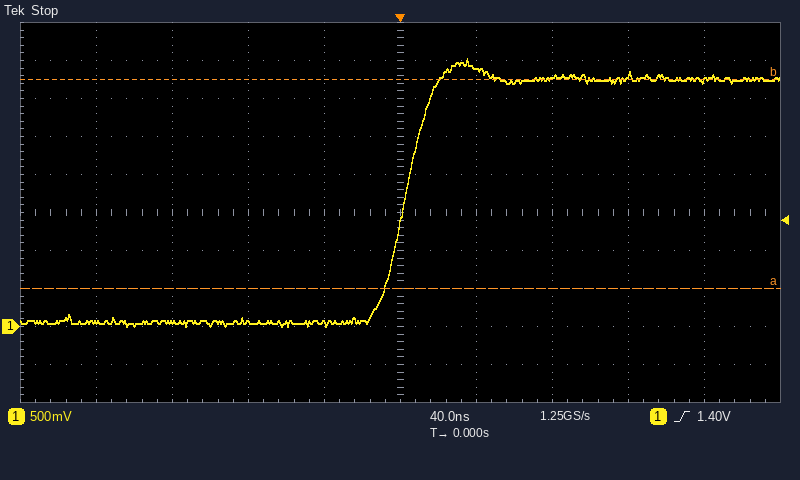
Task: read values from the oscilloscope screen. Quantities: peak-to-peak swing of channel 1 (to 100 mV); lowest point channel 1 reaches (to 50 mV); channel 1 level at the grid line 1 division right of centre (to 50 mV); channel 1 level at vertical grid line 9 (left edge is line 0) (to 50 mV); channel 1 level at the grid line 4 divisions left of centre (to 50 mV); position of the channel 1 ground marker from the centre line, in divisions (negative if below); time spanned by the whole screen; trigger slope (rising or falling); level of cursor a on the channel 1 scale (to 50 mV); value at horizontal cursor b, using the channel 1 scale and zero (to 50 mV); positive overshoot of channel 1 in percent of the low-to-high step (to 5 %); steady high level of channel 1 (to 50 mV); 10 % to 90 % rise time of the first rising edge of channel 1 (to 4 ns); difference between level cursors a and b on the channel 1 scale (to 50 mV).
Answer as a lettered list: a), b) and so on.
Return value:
a) 3.50 V
b) 0 mV
c) 3.40 V
d) 3.25 V
e) 50 mV
f) -3.0 div
g) 400 ns
h) rising
i) 500 mV
j) 3.25 V
k) 10 %
l) 3.25 V
m) 24 ns
n) 2.75 V
